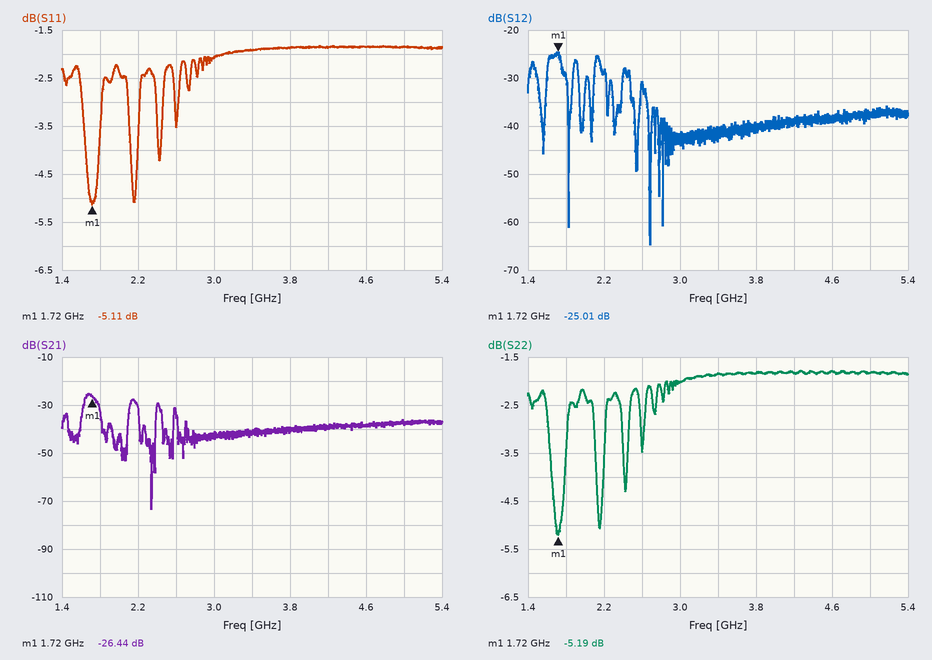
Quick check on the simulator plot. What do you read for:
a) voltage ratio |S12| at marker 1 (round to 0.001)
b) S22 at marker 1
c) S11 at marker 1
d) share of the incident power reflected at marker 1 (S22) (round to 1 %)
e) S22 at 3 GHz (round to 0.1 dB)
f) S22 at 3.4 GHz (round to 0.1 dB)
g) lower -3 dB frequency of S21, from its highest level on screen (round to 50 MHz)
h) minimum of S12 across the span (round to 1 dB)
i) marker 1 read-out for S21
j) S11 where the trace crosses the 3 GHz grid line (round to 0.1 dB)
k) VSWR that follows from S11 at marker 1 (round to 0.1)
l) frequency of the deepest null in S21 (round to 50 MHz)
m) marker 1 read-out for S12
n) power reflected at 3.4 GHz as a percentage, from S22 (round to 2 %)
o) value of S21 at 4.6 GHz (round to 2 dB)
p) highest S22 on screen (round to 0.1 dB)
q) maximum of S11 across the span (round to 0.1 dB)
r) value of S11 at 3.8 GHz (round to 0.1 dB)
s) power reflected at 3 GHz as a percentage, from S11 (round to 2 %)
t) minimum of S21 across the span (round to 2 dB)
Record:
0.056
-5.19 dB
-5.11 dB
30 %
-2.0 dB
-1.8 dB
1.65 GHz
-65 dB
-26.44 dB
-2.1 dB
3.5
2.35 GHz
-25.01 dB
66 %
-38 dB
-1.8 dB
-1.8 dB
-1.9 dB
62 %
-74 dB
